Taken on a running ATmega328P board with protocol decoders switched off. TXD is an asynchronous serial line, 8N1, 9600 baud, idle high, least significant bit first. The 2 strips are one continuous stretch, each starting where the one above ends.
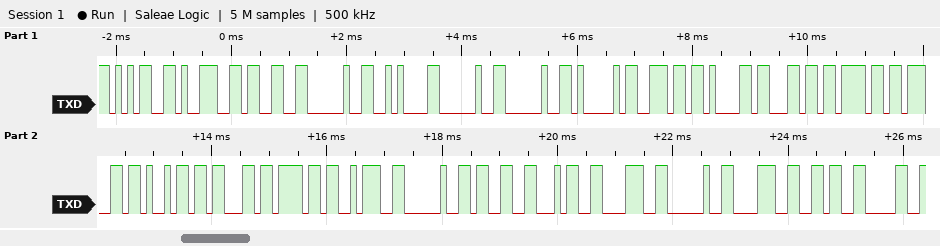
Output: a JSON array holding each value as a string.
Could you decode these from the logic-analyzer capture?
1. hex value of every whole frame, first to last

["0x35 0x39 0x33 0x20 0x0A 0x20 0x20 0x41 0x6E 0x61 0x6C 0x6F 0x67 0x69 0x63 0x6F 0x3A 0x20 0x33 0x34 0x38 0x20 0x38 0x36 0x30"]
